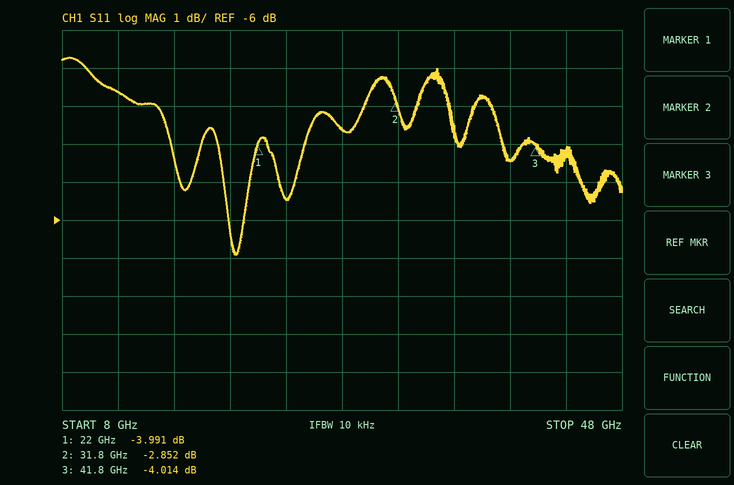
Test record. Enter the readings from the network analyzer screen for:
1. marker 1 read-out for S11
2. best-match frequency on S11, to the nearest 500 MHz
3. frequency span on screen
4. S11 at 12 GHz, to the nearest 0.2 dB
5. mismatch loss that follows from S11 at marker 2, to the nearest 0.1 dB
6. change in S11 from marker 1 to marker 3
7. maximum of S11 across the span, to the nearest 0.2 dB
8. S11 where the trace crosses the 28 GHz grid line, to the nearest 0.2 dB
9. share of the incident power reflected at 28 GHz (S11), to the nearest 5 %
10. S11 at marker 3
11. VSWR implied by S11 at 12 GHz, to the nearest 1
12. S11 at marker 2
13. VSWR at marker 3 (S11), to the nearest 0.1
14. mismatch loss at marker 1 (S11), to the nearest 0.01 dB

-3.991 dB
20.5 GHz
40 GHz
-2.6 dB
3.2 dB
-0.023 dB
-1.8 dB
-3.6 dB
45 %
-4.014 dB
7
-2.852 dB
4.4
2.21 dB
